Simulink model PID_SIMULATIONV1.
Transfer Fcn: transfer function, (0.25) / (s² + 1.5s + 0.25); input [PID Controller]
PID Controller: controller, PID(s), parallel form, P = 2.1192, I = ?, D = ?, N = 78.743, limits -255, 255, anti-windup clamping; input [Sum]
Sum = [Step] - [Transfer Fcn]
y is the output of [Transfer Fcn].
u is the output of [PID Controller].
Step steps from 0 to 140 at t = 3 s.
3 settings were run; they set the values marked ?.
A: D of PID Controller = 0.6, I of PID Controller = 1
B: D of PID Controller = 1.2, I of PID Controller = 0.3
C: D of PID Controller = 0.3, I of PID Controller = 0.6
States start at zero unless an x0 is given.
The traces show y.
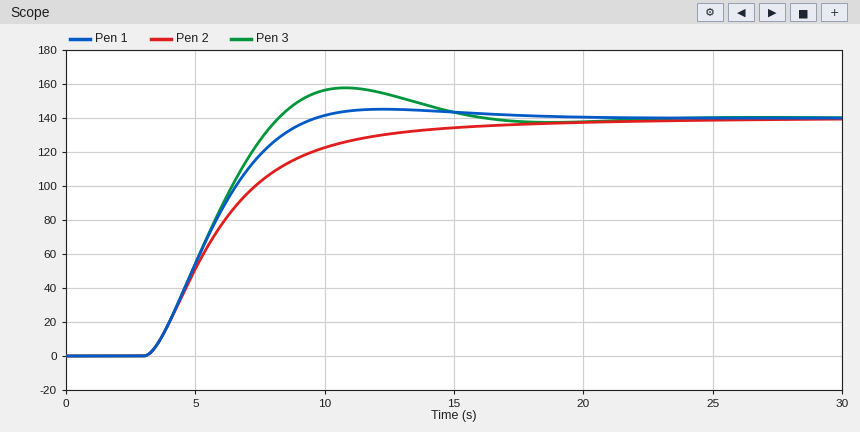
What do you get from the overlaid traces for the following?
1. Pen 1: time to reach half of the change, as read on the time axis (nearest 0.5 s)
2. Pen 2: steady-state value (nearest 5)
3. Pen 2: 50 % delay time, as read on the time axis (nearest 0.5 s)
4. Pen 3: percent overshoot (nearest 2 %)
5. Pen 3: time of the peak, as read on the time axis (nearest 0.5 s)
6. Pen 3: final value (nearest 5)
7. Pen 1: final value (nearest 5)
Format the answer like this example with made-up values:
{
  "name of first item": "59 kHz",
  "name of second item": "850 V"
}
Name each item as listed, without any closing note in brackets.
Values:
{
  "Pen 1: time to reach half of the change, as read on the time axis": "5.5 s",
  "Pen 2: steady-state value": "140",
  "Pen 2: 50 % delay time, as read on the time axis": "5.5 s",
  "Pen 3: percent overshoot": "12 %",
  "Pen 3: time of the peak, as read on the time axis": "11.0 s",
  "Pen 3: final value": "140",
  "Pen 1: final value": "140"
}
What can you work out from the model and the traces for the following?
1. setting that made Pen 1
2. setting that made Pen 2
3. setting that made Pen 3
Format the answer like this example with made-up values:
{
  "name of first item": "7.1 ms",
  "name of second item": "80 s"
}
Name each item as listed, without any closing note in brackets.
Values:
{
  "setting that made Pen 1": "C",
  "setting that made Pen 2": "B",
  "setting that made Pen 3": "A"
}
